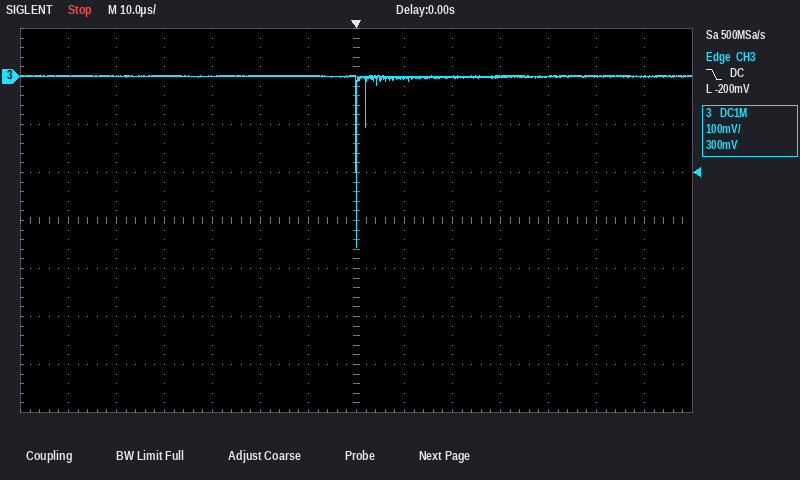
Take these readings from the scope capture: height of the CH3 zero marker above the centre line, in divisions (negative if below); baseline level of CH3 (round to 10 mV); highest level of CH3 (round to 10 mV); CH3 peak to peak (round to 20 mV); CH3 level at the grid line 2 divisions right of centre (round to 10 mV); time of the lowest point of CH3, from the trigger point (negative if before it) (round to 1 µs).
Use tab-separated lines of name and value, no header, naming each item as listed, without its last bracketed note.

height of the CH3 zero marker above the centre line, in divisions	+3.0 div
baseline level of CH3	0 mV
highest level of CH3	0 mV
CH3 peak to peak	360 mV
CH3 level at the grid line 2 divisions right of centre	0 mV
time of the lowest point of CH3, from the trigger point (negative if before it)	0 µs
